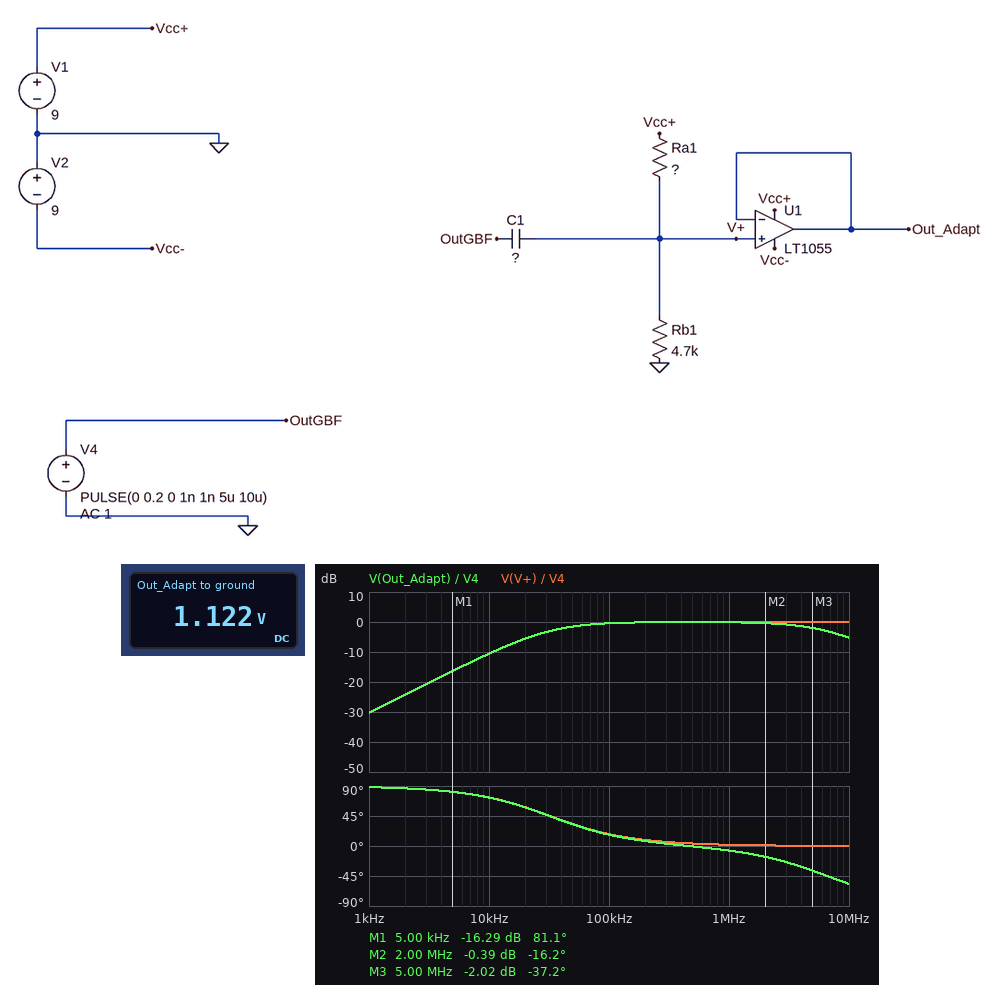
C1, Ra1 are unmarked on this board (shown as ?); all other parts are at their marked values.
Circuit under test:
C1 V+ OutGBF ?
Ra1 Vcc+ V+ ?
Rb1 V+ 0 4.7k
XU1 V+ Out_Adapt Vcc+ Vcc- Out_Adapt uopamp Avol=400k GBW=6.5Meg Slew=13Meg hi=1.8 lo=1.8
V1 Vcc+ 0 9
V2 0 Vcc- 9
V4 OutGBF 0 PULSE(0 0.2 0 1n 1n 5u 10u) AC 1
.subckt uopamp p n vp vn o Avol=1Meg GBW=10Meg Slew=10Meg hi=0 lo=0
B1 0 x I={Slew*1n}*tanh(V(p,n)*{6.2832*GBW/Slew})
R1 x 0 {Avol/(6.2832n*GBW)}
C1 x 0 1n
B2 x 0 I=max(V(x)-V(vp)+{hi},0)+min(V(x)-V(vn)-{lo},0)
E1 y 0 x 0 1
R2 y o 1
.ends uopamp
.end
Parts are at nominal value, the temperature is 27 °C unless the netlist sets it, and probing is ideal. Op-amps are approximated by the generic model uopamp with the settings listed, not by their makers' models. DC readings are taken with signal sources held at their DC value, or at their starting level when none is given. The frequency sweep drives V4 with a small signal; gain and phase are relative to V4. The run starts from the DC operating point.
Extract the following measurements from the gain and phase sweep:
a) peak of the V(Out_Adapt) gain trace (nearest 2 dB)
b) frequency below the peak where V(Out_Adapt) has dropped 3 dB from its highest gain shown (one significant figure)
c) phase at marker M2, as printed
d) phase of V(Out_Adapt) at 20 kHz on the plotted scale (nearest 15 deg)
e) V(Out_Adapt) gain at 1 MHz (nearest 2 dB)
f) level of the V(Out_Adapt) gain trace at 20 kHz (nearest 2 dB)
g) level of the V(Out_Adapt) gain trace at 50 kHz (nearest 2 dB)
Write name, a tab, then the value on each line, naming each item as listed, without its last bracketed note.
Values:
peak of the V(Out_Adapt) gain trace	0 dB
frequency below the peak where V(Out_Adapt) has dropped 3 dB from its highest gain shown	30 kHz
phase at marker M2, as printed	-16.2 deg
phase of V(Out_Adapt) at 20 kHz on the plotted scale	60 deg
V(Out_Adapt) gain at 1 MHz	0 dB
level of the V(Out_Adapt) gain trace at 20 kHz	-6 dB
level of the V(Out_Adapt) gain trace at 50 kHz	-2 dB
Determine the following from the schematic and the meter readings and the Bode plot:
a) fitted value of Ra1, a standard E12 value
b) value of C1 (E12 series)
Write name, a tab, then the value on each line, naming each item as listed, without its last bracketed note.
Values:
fitted value of Ra1, a standard E12 value	33 kΩ
value of C1	1.2 nF
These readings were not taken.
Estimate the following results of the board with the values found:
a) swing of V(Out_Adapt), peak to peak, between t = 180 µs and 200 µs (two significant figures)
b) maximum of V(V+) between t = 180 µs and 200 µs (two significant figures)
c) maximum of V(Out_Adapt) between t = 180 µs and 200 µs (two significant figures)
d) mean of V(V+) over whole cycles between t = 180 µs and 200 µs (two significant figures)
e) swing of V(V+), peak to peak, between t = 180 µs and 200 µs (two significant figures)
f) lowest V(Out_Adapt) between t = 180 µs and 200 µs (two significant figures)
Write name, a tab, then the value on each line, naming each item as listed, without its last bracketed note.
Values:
swing of V(Out_Adapt), peak to peak, between t = 180 µs and 200 µs	290 mV
maximum of V(V+) between t = 180 µs and 200 µs	1.3 V
maximum of V(Out_Adapt) between t = 180 µs and 200 µs	1.3 V
mean of V(V+) over whole cycles between t = 180 µs and 200 µs	1.1 V
swing of V(V+), peak to peak, between t = 180 µs and 200 µs	290 mV
lowest V(Out_Adapt) between t = 180 µs and 200 µs	980 mV
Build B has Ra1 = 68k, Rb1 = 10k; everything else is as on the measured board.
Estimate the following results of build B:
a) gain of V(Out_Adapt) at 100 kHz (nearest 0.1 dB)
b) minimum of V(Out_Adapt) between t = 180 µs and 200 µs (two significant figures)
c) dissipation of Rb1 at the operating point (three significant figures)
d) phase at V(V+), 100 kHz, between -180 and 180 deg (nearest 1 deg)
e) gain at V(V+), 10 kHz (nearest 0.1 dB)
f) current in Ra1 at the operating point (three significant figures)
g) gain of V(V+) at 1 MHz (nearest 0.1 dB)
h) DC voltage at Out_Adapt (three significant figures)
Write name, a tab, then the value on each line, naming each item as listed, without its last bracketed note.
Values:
gain of V(Out_Adapt) at 100 kHz	-0.1 dB
minimum of V(Out_Adapt) between t = 180 µs and 200 µs	1.0 V
dissipation of Rb1 at the operating point	133 µW
phase at V(V+), 100 kHz, between -180 and 180 deg	9 deg
gain at V(V+), 10 kHz	-5.2 dB
current in Ra1 at the operating point	115 µA
gain of V(V+) at 1 MHz	0 dB
DC voltage at Out_Adapt	1.15 V
